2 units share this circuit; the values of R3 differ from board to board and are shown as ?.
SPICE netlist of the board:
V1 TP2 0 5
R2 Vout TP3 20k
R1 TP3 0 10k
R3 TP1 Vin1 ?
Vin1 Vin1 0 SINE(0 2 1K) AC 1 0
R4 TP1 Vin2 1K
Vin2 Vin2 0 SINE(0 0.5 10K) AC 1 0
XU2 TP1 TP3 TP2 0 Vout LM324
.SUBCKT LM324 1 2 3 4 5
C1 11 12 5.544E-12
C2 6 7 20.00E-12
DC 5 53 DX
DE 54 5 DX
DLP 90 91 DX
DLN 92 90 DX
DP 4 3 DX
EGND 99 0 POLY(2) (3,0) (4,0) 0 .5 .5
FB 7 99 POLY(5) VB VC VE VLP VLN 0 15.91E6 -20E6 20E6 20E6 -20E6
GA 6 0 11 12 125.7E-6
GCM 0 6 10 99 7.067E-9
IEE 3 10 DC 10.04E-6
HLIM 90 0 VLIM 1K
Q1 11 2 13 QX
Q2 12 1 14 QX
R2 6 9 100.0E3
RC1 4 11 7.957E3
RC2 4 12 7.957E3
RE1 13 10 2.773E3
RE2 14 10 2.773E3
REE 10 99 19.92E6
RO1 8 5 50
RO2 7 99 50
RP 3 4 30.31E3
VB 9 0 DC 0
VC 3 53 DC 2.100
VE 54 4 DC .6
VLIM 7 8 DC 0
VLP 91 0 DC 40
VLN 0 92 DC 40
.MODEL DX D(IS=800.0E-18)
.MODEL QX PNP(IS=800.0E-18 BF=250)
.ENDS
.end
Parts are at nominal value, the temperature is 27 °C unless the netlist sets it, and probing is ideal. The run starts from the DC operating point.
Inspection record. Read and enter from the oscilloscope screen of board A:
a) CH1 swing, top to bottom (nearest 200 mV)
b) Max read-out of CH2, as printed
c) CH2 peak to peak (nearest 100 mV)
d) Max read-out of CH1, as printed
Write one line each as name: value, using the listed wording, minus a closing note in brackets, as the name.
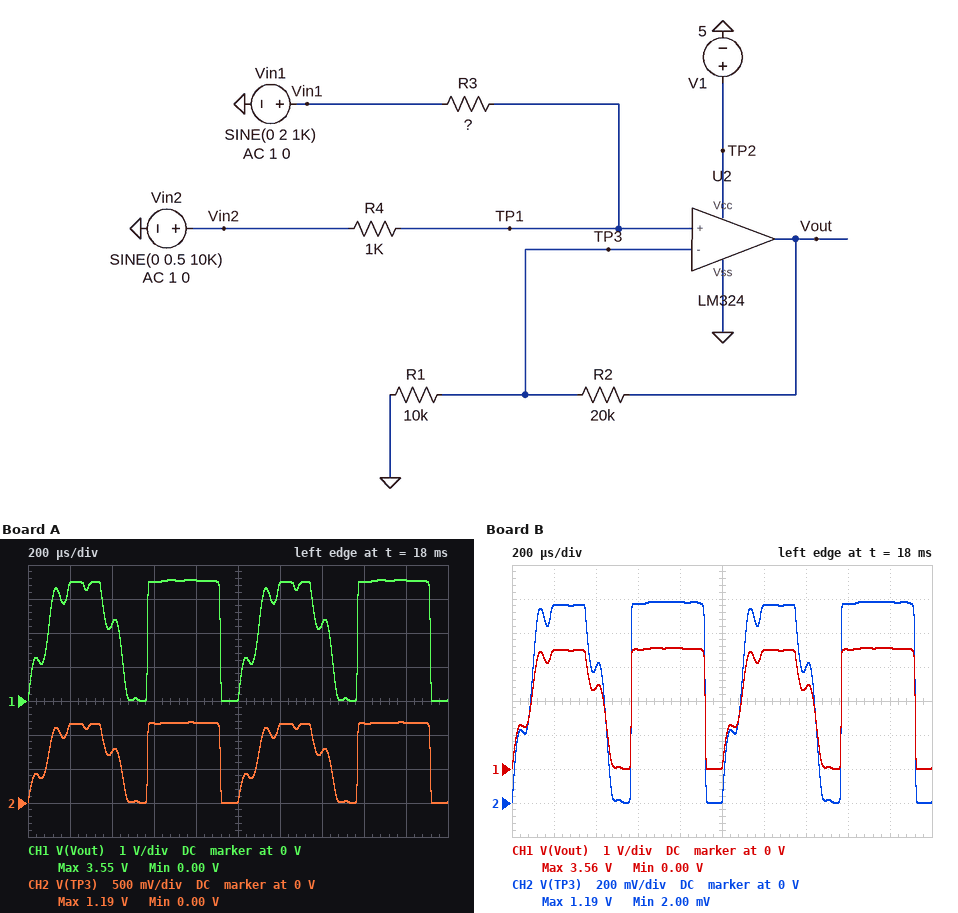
CH1 swing, top to bottom: 3.6 V
Max read-out of CH2, as printed: 1.19 V
CH2 peak to peak: 1.2 V
Max read-out of CH1, as printed: 3.55 V
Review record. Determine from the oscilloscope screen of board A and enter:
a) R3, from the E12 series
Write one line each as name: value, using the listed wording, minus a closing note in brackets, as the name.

R3, from the E12 series: 560 Ω
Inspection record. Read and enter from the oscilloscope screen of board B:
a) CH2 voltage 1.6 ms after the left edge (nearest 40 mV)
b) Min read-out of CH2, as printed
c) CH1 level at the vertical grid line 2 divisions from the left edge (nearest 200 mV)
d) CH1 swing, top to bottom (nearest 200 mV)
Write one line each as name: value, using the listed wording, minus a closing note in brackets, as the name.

CH2 voltage 1.6 ms after the left edge: 1.16 V
Min read-out of CH2, as printed: 2.00 mV
CH1 level at the vertical grid line 2 divisions from the left edge: 2.4 V
CH1 swing, top to bottom: 3.6 V
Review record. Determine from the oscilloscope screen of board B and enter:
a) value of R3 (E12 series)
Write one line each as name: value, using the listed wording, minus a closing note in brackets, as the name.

value of R3: 470 Ω
